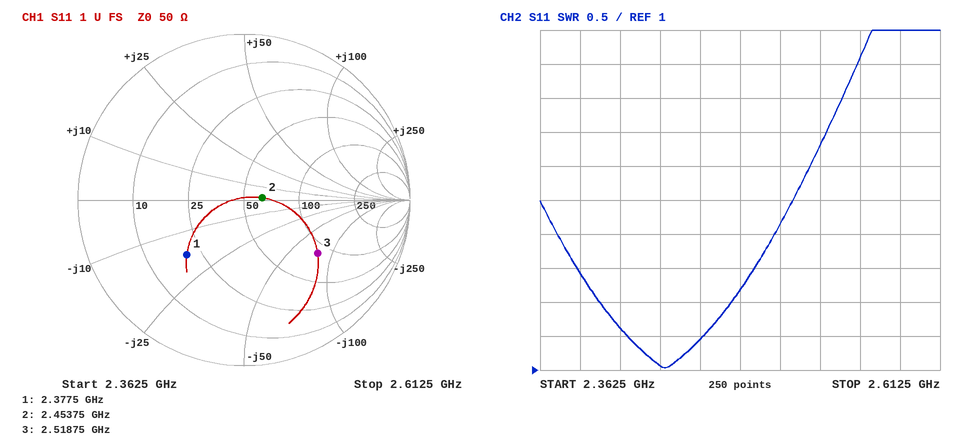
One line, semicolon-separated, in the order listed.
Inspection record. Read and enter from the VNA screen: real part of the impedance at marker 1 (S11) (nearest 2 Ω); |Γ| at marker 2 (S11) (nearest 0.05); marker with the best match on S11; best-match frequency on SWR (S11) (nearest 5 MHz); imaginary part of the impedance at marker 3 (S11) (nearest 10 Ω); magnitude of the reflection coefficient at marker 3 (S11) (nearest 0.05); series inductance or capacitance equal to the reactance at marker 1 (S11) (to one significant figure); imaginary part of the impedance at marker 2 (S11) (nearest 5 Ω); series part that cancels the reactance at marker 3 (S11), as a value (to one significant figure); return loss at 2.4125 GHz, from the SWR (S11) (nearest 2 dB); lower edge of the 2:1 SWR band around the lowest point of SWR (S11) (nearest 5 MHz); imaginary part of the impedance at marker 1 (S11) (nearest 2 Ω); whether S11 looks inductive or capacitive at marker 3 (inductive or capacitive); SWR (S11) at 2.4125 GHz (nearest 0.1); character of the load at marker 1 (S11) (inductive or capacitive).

20 Ω; 0.10; marker 2; 2.440 GHz; -80 Ω; 0.55; 4 pF; 0 Ω; 5 nH; 12 dB; 2.400 GHz; -18 Ω; capacitive; 1.6; capacitive
